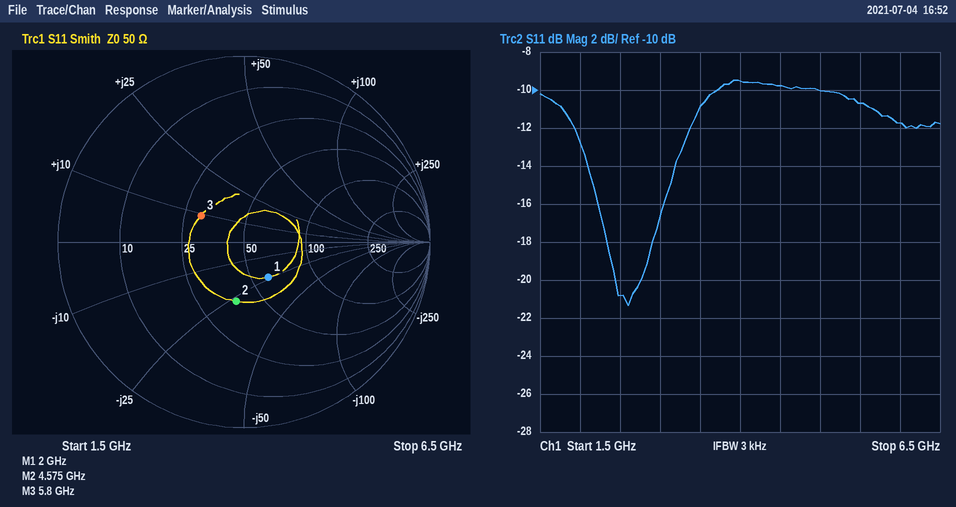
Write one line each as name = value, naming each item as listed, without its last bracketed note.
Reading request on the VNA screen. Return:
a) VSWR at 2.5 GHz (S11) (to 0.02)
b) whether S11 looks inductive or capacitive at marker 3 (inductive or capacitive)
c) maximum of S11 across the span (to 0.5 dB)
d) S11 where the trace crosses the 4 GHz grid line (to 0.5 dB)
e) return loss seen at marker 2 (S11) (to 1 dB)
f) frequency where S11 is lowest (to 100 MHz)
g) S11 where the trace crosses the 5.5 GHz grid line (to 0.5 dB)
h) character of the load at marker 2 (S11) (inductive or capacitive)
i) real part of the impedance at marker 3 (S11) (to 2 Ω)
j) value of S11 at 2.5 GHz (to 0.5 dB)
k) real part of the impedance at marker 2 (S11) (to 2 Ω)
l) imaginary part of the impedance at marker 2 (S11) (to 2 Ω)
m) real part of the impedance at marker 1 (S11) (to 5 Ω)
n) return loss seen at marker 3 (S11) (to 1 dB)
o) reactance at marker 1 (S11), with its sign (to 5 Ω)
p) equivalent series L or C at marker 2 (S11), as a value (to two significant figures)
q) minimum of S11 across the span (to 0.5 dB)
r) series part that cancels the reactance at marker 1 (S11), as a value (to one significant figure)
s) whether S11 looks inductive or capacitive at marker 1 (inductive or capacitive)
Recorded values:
VSWR at 2.5 GHz (S11) = 1.20
whether S11 looks inductive or capacitive at marker 3 = inductive
maximum of S11 across the span = -9.5 dB
S11 where the trace crosses the 4 GHz grid line = -9.5 dB
return loss seen at marker 2 (S11) = 10 dB
frequency where S11 is lowest = 2.6 GHz
S11 where the trace crosses the 5.5 GHz grid line = -10.5 dB
character of the load at marker 2 (S11) = capacitive
real part of the impedance at marker 3 (S11) = 30 Ω
value of S11 at 2.5 GHz = -21.0 dB
real part of the impedance at marker 2 (S11) = 38 Ω
imaginary part of the impedance at marker 2 (S11) = -26 Ω
real part of the impedance at marker 1 (S11) = 60 Ω
return loss seen at marker 3 (S11) = 11 dB
reactance at marker 1 (S11), with its sign = -25 Ω
equivalent series L or C at marker 2 (S11), as a value = 1.3 pF
minimum of S11 across the span = -21.5 dB
series part that cancels the reactance at marker 1 (S11), as a value = 2 nH
whether S11 looks inductive or capacitive at marker 1 = capacitive
